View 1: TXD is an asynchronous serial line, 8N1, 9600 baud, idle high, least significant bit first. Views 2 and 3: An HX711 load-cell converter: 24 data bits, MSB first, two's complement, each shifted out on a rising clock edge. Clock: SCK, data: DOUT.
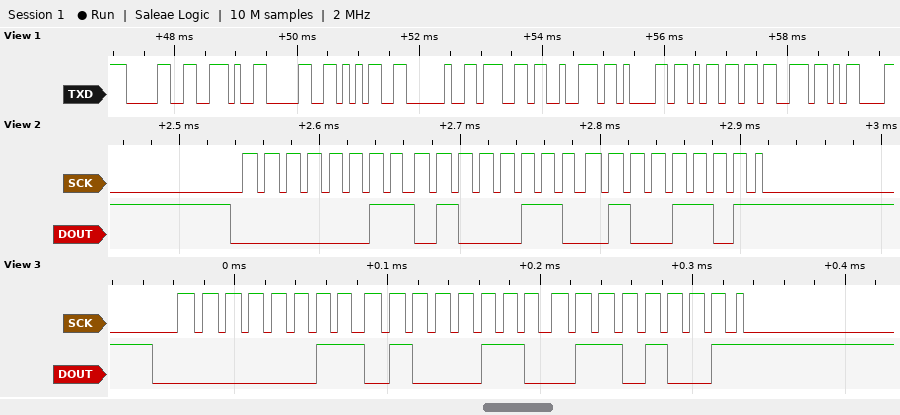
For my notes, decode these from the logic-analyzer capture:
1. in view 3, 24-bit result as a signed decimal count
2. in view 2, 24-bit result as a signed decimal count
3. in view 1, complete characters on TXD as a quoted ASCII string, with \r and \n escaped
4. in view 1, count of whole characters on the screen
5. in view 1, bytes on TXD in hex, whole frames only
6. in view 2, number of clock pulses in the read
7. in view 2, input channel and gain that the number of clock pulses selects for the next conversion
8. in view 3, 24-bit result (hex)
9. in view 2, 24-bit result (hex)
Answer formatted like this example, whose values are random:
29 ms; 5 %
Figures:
214633; 214605; "0.05 grams\r"; 11; 30 2E 30 35 20 67 72 61 6D 73 0D; 25; channel A, gain 128; 0x034669; 0x03464D
